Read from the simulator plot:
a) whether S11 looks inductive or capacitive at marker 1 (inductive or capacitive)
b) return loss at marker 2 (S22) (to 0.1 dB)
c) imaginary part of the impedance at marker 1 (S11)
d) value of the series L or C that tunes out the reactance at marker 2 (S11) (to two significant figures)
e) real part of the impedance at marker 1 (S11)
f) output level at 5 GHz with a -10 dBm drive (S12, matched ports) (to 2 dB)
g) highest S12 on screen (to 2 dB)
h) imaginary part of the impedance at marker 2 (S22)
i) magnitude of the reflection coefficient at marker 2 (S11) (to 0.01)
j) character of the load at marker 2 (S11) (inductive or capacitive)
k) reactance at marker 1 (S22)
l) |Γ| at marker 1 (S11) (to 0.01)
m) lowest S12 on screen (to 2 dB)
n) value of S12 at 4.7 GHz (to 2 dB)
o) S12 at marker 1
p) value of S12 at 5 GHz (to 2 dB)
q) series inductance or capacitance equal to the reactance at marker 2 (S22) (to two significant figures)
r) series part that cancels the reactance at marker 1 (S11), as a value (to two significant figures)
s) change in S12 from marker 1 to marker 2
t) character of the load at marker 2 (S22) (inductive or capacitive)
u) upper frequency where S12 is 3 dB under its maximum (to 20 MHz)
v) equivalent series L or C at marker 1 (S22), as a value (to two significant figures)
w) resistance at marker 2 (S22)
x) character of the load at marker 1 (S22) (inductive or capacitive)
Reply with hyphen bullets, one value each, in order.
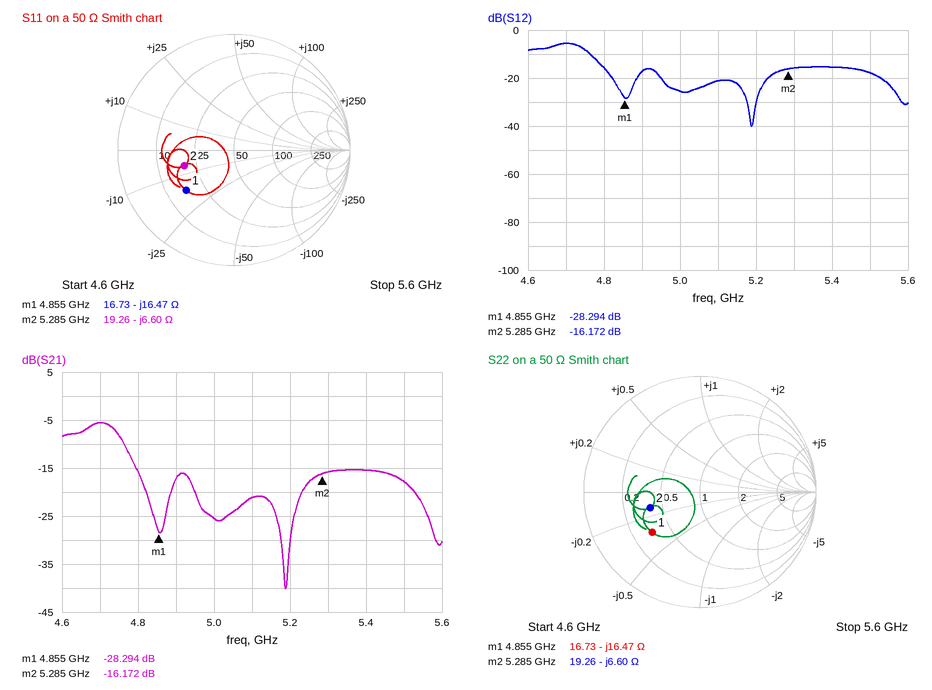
- capacitive
- 6.9 dB
- -16.47 Ω
- 200 pH
- 16.73 Ω
- -36 dBm
- -6 dB
- -6.60 Ω
- 0.45
- capacitive
- -16.47 Ω
- 0.54
- -40 dB
- -6 dB
- -28.294 dB
- -26 dB
- 4.6 pF
- 540 pH
- 12.122 dB
- capacitive
- 4.76 GHz
- 2.0 pF
- 19.26 Ω
- capacitive
